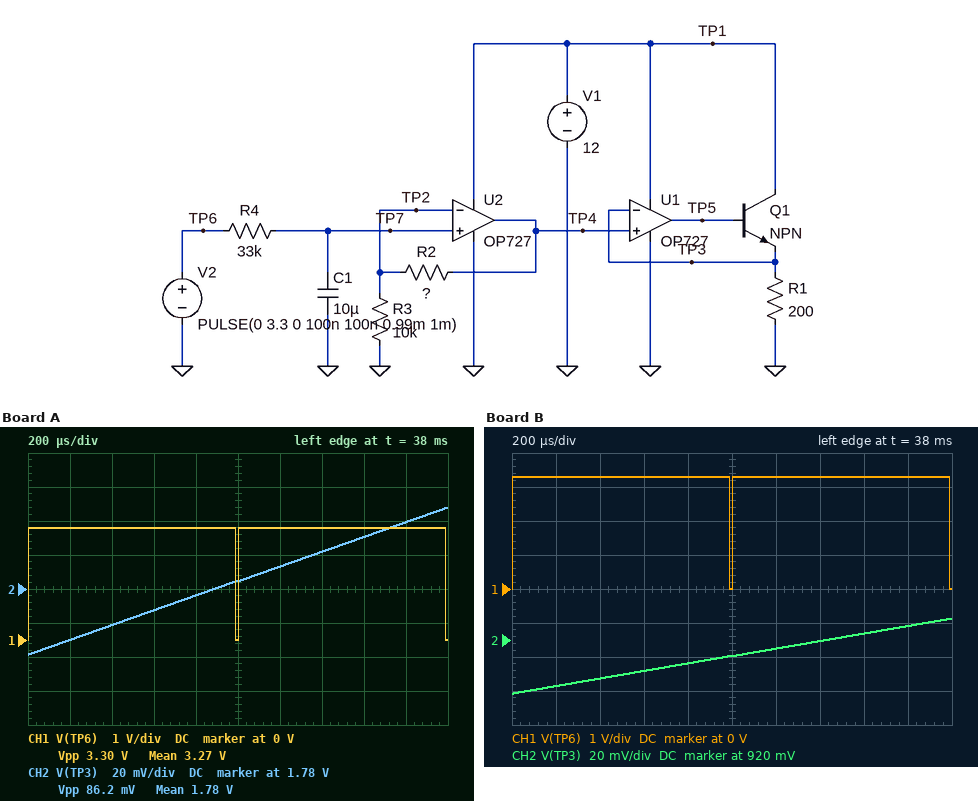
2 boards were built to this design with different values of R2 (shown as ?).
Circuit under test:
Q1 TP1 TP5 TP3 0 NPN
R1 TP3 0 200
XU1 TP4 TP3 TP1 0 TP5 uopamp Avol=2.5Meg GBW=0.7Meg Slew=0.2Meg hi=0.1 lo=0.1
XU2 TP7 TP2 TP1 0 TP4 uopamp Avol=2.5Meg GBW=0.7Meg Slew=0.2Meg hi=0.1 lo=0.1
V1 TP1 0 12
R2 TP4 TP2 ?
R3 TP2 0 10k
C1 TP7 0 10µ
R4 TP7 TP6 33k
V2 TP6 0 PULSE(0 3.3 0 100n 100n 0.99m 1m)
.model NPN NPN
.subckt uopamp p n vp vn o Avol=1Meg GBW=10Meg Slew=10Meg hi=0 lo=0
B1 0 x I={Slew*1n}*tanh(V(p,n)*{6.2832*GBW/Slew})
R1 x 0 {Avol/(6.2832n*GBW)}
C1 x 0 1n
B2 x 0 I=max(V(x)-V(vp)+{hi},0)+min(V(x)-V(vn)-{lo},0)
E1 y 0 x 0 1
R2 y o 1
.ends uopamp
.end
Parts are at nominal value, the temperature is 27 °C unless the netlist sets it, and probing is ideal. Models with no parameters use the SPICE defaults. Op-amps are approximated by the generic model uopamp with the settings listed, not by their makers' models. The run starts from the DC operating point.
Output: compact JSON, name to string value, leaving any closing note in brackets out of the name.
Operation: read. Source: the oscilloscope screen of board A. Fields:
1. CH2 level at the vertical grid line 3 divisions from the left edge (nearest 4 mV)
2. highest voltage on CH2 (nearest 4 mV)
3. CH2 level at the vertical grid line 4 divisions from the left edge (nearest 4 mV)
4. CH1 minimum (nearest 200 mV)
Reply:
{"CH2 level at the vertical grid line 3 divisions from the left edge": "1.768 V", "highest voltage on CH2": "1.828 V", "CH2 level at the vertical grid line 4 divisions from the left edge": "1.776 V", "CH1 minimum": "0 V"}
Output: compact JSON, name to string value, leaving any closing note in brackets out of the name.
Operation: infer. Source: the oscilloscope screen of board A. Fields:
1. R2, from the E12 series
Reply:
{"R2, from the E12 series": "39 kΩ"}
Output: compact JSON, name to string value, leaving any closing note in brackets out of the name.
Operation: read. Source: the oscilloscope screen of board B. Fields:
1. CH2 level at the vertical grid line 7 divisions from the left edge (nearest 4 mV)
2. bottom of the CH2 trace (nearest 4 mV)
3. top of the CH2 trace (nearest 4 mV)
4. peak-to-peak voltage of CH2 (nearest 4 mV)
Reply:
{"CH2 level at the vertical grid line 7 divisions from the left edge": "920 mV", "bottom of the CH2 trace": "888 mV", "top of the CH2 trace": "932 mV", "peak-to-peak voltage of CH2": "44 mV"}
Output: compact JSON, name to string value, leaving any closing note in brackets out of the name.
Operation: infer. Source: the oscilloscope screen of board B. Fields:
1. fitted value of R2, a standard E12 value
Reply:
{"fitted value of R2, a standard E12 value": "15 kΩ"}
